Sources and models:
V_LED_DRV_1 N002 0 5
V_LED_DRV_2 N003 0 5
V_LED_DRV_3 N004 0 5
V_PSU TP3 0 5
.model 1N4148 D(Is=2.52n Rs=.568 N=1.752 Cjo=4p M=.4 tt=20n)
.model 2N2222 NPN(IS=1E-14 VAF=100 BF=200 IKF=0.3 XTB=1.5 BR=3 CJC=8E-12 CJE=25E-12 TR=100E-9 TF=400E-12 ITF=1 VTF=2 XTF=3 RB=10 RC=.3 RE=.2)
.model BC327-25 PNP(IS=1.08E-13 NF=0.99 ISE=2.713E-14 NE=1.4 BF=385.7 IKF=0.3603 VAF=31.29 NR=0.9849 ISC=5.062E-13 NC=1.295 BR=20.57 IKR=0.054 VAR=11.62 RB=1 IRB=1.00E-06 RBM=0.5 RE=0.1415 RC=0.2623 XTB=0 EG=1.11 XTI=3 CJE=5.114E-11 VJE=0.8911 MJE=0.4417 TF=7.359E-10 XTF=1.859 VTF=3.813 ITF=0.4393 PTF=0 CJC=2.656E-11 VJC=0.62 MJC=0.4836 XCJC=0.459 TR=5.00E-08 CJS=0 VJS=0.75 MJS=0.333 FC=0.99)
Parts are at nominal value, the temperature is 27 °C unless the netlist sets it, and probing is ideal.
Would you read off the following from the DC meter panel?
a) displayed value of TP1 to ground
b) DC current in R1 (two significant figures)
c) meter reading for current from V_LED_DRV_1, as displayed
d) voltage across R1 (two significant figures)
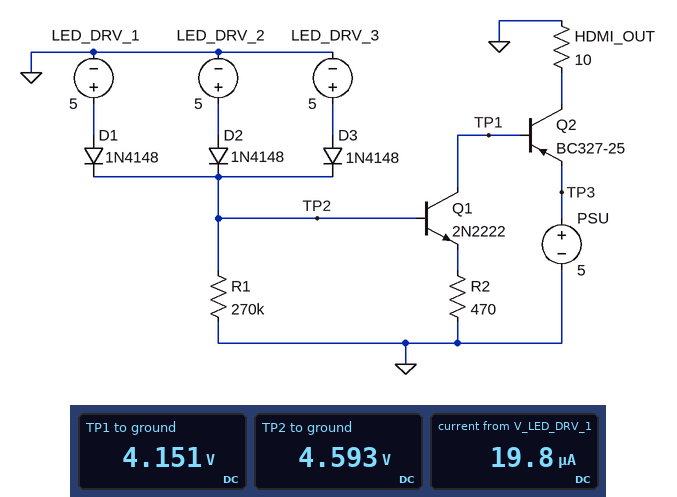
4.151 V
17 µA
19.8 µA
4.6 V
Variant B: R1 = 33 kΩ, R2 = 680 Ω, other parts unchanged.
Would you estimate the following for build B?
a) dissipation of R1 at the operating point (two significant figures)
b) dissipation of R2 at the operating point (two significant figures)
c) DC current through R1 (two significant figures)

630 µW
22 mW
140 µA
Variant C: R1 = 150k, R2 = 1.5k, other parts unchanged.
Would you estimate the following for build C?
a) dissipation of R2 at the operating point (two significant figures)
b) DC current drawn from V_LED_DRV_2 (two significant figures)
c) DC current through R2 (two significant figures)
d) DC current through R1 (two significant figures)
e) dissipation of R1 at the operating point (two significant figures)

10 mW
15 µA
2.6 mA
31 µA
140 µW
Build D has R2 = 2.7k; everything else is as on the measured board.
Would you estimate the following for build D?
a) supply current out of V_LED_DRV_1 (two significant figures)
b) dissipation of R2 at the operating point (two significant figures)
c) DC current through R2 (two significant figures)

8.2 µA
5.8 mW
1.5 mA
